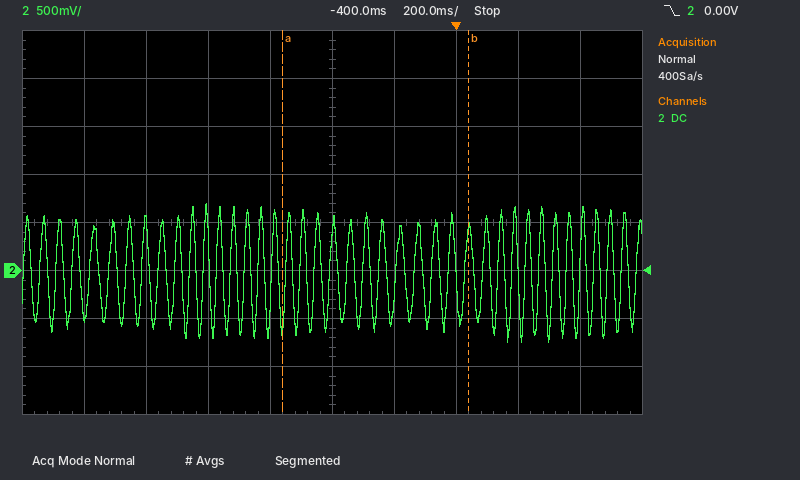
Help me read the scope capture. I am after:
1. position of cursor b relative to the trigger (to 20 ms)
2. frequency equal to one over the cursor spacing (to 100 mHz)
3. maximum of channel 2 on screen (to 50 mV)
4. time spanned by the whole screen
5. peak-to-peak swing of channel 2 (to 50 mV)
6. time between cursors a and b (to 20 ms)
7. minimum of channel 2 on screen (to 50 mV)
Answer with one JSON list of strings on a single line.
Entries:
["+40 ms", "1.7 Hz", "700 mV", "2 s", "1.45 V", "600 ms", "-750 mV"]
